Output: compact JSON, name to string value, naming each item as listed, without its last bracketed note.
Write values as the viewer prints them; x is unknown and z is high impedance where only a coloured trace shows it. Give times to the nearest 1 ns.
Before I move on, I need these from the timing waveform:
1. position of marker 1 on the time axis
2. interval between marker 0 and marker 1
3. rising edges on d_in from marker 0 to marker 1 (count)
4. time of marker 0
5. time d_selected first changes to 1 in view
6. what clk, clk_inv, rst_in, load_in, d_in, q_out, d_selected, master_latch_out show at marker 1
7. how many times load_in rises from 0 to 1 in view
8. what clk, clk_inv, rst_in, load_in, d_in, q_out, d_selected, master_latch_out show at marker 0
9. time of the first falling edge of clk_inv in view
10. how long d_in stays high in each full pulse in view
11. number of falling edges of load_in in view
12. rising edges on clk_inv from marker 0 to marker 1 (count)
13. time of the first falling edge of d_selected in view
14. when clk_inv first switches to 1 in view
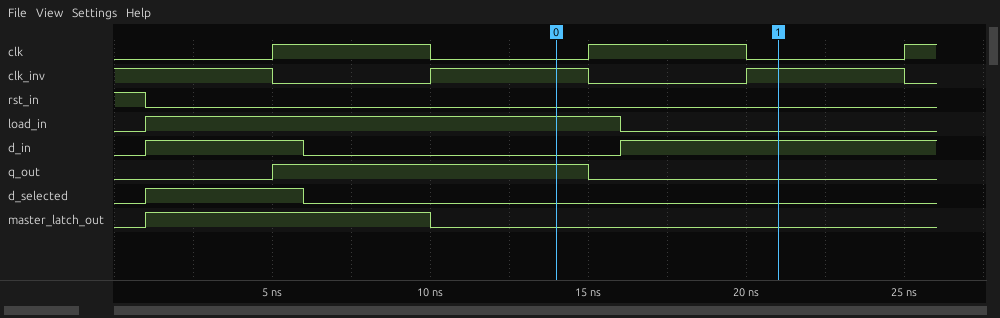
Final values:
{"position of marker 1 on the time axis": "21 ns", "interval between marker 0 and marker 1": "7 ns", "rising edges on d_in from marker 0 to marker 1": "1", "time of marker 0": "14 ns", "time d_selected first changes to 1 in view": "1 ns", "what clk, clk_inv, rst_in, load_in, d_in, q_out, d_selected, master_latch_out show at marker 1": "clk=0, clk_inv=1, rst_in=0, load_in=0, d_in=1, q_out=0, d_selected=0, master_latch_out=0", "how many times load_in rises from 0 to 1 in view": "1", "what clk, clk_inv, rst_in, load_in, d_in, q_out, d_selected, master_latch_out show at marker 0": "clk=0, clk_inv=1, rst_in=0, load_in=1, d_in=0, q_out=1, d_selected=0, master_latch_out=0", "time of the first falling edge of clk_inv in view": "5 ns", "how long d_in stays high in each full pulse in view": "5 ns", "number of falling edges of load_in in view": "1", "rising edges on clk_inv from marker 0 to marker 1": "1", "time of the first falling edge of d_selected in view": "6 ns", "when clk_inv first switches to 1 in view": "10 ns"}
